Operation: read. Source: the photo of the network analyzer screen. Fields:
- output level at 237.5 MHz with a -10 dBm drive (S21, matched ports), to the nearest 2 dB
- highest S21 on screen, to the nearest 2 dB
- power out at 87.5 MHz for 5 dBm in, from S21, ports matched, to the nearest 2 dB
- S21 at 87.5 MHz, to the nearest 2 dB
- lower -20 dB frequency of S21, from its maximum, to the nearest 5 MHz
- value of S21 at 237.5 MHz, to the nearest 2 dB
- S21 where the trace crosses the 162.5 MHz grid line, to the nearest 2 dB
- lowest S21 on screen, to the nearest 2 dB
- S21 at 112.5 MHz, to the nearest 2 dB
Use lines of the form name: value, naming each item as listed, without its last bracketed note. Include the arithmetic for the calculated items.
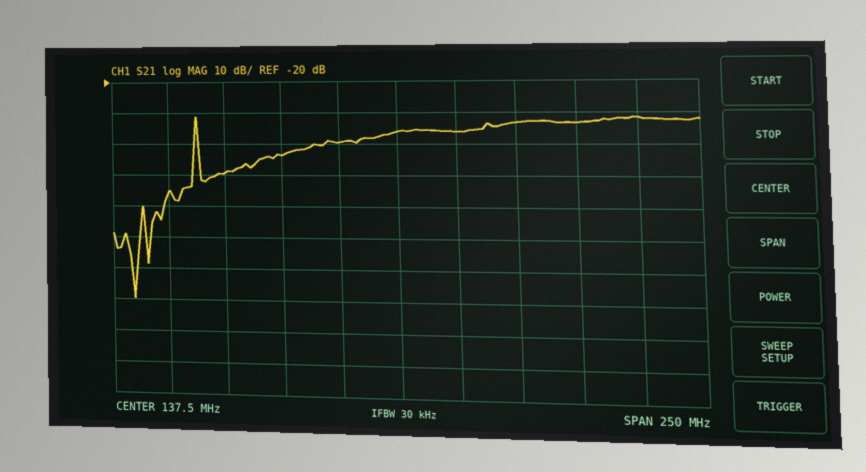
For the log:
output level at 237.5 MHz with a -10 dBm drive (S21, matched ports), to the nearest 2 dB: -10 dBm + (-32 dB) = -42 dBm
highest S21 on screen, to the nearest 2 dB: -32 dB
power out at 87.5 MHz for 5 dBm in, from S21, ports matched, to the nearest 2 dB: 5 dBm + (-44 dB) = -38 dBm
S21 at 87.5 MHz, to the nearest 2 dB: -44 dB
lower -20 dB frequency of S21, from its maximum, to the nearest 5 MHz: 50 MHz
value of S21 at 237.5 MHz, to the nearest 2 dB: -32 dB
S21 where the trace crosses the 162.5 MHz grid line, to the nearest 2 dB: -36 dB
lowest S21 on screen, to the nearest 2 dB: -90 dB
S21 at 112.5 MHz, to the nearest 2 dB: -40 dB
